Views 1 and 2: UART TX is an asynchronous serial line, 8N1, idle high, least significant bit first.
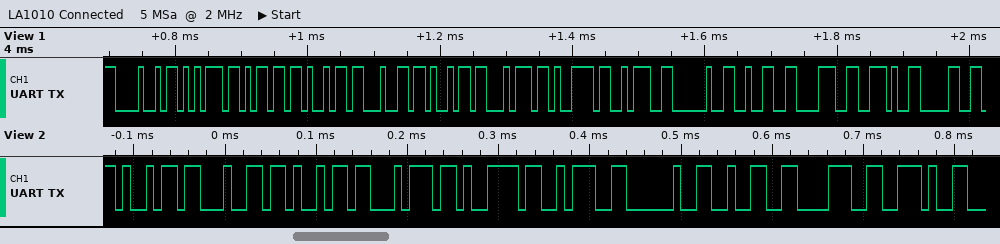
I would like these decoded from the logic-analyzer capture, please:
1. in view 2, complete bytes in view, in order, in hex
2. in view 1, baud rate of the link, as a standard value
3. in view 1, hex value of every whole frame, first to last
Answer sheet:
69 64 69 74 79 3A 20 32 38 2E
115200 baud
48 75 6D 69 64 69 74 79 3A 20 32 38 2E 30
